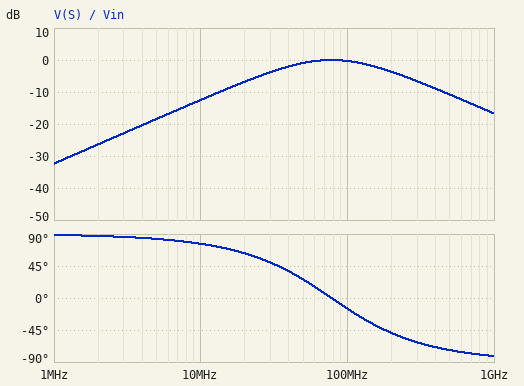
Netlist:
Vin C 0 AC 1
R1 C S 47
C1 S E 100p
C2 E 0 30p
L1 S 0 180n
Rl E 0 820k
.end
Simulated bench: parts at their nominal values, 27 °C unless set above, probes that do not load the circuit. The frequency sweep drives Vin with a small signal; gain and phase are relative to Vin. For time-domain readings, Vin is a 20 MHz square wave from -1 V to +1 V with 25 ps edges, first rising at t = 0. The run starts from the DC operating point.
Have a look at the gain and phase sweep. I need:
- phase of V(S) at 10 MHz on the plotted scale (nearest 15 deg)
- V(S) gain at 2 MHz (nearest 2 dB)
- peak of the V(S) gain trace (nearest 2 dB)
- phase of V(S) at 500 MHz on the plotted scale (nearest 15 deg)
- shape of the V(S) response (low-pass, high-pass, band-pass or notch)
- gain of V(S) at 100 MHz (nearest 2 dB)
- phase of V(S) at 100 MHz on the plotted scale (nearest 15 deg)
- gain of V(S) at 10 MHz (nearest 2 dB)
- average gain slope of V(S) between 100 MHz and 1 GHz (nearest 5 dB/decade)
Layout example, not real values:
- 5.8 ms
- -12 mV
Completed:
- 75 deg
- -26 dB
- 0 dB
- -75 deg
- band-pass
- 0 dB
- -15 deg
- -12 dB
- -15 dB/decade
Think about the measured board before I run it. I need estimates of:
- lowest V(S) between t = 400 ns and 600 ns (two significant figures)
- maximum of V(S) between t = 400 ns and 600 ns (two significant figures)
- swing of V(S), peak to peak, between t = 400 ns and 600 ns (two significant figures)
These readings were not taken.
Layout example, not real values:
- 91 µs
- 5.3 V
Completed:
- -1.4 V
- 1.4 V
- 2.9 V
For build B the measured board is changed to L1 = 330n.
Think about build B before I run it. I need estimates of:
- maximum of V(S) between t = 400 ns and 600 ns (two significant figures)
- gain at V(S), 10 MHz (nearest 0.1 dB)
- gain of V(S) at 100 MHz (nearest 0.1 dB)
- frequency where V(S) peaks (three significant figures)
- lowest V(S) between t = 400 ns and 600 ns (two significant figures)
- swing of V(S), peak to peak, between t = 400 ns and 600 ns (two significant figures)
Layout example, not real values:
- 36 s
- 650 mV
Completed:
- 1.6 V
- -7.7 dB
- -0.8 dB
- 57.7 MHz
- -1.6 V
- 3.1 V
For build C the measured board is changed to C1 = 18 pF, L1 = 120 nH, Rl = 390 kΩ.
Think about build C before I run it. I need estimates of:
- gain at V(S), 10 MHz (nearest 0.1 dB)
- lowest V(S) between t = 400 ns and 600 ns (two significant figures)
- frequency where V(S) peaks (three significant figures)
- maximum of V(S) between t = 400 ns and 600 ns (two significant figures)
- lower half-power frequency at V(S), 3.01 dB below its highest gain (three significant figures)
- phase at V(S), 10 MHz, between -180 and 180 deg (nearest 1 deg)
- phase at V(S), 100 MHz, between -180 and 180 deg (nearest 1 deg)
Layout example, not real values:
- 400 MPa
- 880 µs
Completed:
- -16.0 dB
- -1.5 V
- 137 MHz
- 1.5 V
- 53.0 MHz
- 81 deg
- 16 deg
